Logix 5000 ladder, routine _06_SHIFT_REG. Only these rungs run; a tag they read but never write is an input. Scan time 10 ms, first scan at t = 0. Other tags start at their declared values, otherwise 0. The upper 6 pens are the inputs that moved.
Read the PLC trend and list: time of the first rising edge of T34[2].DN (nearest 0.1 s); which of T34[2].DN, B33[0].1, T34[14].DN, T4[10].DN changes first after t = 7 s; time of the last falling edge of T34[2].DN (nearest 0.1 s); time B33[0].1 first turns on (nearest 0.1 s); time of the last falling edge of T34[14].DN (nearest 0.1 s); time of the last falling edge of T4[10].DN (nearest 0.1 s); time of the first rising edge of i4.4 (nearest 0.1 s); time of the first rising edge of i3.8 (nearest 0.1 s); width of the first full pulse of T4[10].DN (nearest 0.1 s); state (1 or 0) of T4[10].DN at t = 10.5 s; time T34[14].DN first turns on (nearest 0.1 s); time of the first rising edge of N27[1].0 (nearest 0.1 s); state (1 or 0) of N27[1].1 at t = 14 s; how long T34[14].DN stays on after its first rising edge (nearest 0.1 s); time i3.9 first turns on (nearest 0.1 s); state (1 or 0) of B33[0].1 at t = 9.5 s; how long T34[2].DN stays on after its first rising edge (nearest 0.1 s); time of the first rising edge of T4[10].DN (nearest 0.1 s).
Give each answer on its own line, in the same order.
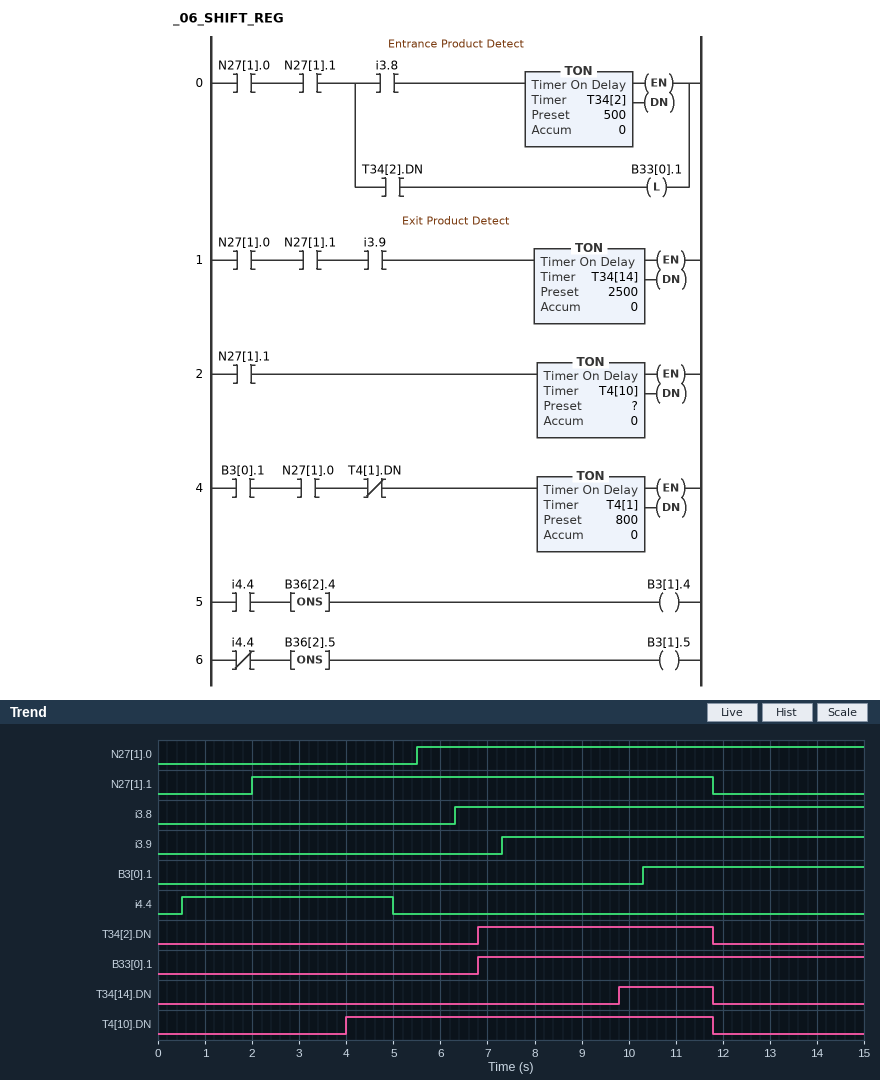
6.8 s
T34[14].DN
11.8 s
6.8 s
11.8 s
11.8 s
0.5 s
6.3 s
7.8 s
1
9.8 s
5.5 s
0
2.0 s
7.3 s
1
5.0 s
4.0 s
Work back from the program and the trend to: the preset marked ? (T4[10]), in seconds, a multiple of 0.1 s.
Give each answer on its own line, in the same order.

2.0 s
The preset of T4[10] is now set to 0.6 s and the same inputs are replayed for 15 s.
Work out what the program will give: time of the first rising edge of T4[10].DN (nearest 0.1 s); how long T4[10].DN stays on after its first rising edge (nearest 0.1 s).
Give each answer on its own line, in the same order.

2.6 s
9.2 s
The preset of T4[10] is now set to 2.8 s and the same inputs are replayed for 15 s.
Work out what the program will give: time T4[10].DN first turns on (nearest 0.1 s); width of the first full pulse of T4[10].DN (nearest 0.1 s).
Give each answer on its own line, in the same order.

4.8 s
7.0 s
